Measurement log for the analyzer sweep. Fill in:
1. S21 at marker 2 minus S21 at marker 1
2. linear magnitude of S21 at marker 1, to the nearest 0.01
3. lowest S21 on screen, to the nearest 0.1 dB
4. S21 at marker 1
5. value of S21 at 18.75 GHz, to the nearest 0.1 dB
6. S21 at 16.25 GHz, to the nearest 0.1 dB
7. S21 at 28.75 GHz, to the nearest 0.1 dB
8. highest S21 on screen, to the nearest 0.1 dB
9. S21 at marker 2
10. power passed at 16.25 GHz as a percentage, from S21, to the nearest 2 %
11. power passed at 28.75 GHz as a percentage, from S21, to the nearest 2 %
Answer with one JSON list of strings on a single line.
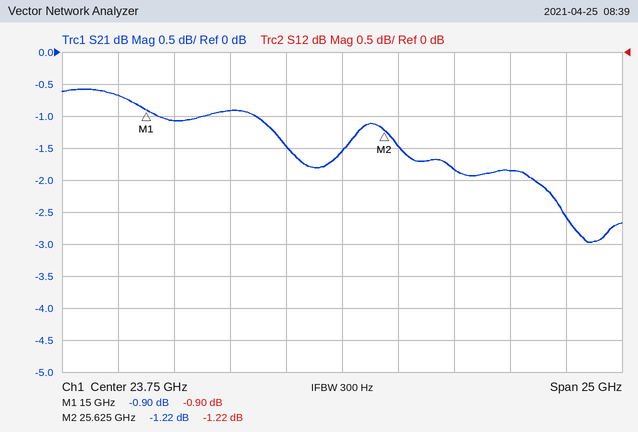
["-0.32 dB", "0.90", "-3.0 dB", "-0.90 dB", "-0.9 dB", "-1.1 dB", "-1.8 dB", "-0.6 dB", "-1.22 dB", "78 %", "66 %"]
